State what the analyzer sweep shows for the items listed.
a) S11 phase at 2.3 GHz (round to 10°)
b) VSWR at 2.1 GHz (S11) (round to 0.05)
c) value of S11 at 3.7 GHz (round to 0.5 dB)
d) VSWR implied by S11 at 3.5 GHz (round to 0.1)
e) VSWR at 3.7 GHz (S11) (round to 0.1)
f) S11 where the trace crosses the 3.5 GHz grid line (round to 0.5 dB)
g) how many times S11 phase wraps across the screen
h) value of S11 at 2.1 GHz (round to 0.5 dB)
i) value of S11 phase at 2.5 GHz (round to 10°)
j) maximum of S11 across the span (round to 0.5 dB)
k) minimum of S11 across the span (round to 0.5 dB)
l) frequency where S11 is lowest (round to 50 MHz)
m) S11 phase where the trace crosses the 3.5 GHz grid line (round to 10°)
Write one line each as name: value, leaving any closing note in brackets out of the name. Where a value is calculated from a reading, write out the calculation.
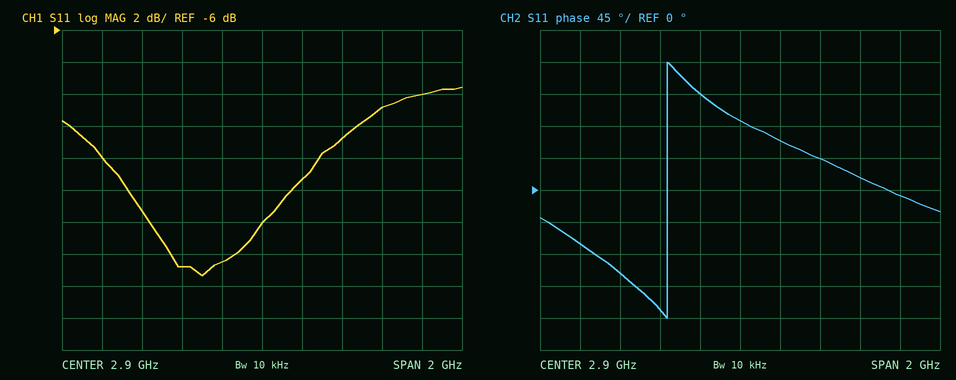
S11 phase at 2.3 GHz: -120°
VSWR at 2.1 GHz (S11): |Γ| = 10^(-14/20) = 0.1995; VSWR = (1 + 0.1995)/(1 − 0.1995) ≈ 1.50
value of S11 at 3.7 GHz: -10.0 dB
VSWR implied by S11 at 3.5 GHz: |Γ| = 10^(-11/20) = 0.2818; VSWR = (1 + 0.2818)/(1 − 0.2818) ≈ 1.8
VSWR at 3.7 GHz (S11): |Γ| = 10^(-10/20) = 0.3162; VSWR = (1 + 0.3162)/(1 − 0.3162) ≈ 1.9
S11 where the trace crosses the 3.5 GHz grid line: -11.0 dB
how many times S11 phase wraps across the screen: 1
value of S11 at 2.1 GHz: -14.0 dB
value of S11 phase at 2.5 GHz: -170°
maximum of S11 across the span: -9.5 dB
minimum of S11 across the span: -21.5 dB
frequency where S11 is lowest: 2.60 GHz
S11 phase where the trace crosses the 3.5 GHz grid line: 20°
